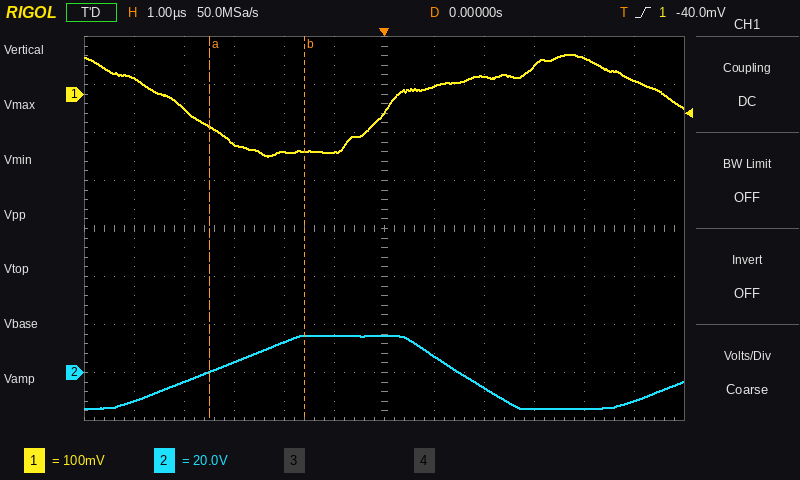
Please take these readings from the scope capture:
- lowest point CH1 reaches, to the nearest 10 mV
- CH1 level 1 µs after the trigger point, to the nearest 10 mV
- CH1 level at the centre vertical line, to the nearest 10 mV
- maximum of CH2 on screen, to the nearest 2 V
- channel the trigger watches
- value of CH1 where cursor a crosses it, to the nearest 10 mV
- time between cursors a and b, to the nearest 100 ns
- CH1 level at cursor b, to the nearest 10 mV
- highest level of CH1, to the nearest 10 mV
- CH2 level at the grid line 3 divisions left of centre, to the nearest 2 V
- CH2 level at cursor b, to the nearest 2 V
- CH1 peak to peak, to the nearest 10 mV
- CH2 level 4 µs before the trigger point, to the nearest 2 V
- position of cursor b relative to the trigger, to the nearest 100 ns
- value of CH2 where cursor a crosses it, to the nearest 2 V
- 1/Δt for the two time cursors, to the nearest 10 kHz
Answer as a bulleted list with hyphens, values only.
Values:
- -130 mV
- 20 mV
- -40 mV
- 16 V
- CH1
- -70 mV
- 1.9 µs
- -120 mV
- 80 mV
- 4 V
- 16 V
- 210 mV
- -4 V
- -1.6 µs
- 0 V
- 530 kHz
